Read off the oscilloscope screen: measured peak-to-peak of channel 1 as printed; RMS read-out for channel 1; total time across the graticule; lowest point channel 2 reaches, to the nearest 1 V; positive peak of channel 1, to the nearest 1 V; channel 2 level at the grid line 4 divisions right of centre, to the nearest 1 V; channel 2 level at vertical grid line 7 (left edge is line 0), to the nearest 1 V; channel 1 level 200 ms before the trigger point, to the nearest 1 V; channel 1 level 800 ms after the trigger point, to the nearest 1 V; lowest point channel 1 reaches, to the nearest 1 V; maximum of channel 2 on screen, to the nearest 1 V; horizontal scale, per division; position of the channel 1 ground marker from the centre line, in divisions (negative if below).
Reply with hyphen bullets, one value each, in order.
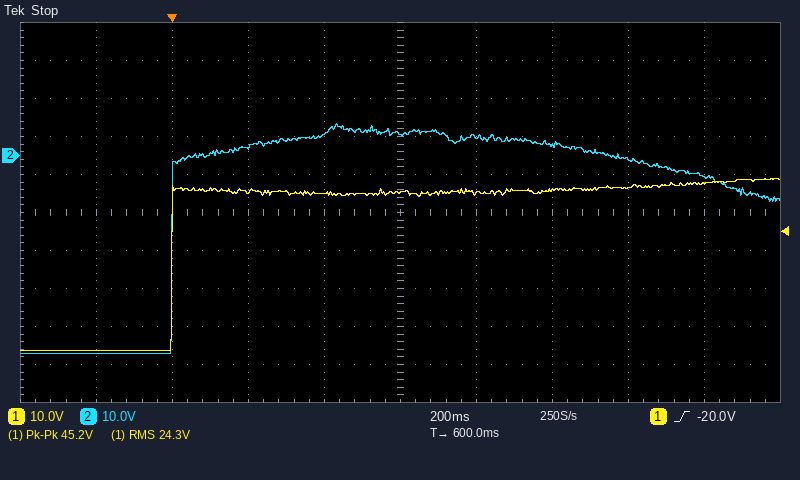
- 45.2 V
- 24.3 V
- 2 s
- -52 V
- -6 V
- -6 V
- 3 V
- -51 V
- -10 V
- -51 V
- 8 V
- 200 ms
- +1.5 div
